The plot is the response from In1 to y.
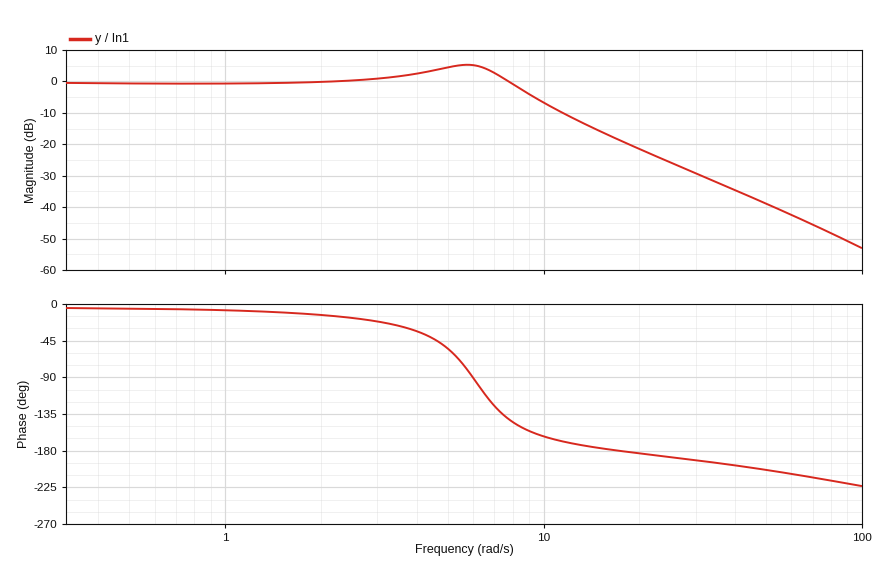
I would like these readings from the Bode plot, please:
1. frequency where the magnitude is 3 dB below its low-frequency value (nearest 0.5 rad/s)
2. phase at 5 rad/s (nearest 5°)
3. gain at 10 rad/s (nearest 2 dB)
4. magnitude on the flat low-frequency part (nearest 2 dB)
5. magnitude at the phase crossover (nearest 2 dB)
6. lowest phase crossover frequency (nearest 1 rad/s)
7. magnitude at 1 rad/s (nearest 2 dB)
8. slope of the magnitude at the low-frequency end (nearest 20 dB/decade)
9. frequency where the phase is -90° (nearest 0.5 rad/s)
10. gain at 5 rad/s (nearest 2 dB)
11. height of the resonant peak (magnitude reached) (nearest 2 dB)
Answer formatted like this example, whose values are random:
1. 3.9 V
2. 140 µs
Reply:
1. 9.0 rad/s
2. -55°
3. -6 dB
4. 0 dB
5. -18 dB
6. 17 rad/s
7. 0 dB
8. 0 dB/decade
9. 6.0 rad/s
10. 4 dB
11. 6 dB
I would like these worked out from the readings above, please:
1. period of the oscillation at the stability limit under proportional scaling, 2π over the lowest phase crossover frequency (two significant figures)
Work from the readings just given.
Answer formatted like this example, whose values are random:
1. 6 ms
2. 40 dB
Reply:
1. 0.37 s
